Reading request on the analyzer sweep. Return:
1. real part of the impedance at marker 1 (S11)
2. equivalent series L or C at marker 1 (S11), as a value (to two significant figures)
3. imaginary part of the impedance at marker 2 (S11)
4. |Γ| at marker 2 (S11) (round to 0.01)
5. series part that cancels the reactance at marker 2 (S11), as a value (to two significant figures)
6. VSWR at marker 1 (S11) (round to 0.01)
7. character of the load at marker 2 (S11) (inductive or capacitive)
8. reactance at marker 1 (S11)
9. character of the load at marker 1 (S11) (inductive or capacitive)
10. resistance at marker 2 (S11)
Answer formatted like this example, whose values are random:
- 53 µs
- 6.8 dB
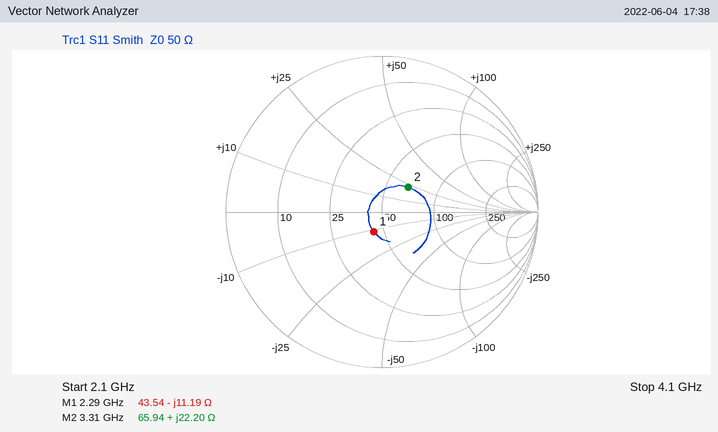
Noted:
- 43.54 Ω
- 6.2 pF
- +22.20 Ω
- 0.23
- 2.2 pF
- 1.32
- inductive
- -11.19 Ω
- capacitive
- 65.94 Ω
